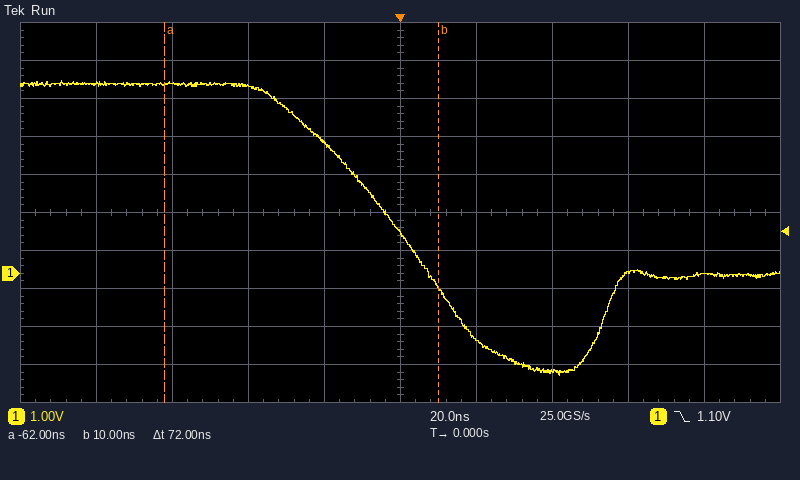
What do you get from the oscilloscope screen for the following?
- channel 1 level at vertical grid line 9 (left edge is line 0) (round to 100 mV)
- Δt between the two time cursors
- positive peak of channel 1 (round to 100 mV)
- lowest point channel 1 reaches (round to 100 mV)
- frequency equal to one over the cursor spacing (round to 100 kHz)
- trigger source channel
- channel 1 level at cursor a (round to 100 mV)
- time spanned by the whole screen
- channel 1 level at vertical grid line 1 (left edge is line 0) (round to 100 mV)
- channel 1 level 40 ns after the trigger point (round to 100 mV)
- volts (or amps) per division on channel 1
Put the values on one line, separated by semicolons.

0.0 V; 72 ns; 5.1 V; -2.7 V; 13.9 MHz; channel 1; 5.0 V; 200 ns; 5.0 V; -2.6 V; 1 V
